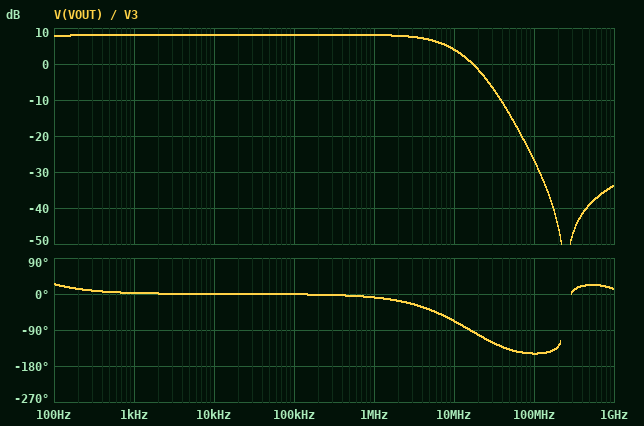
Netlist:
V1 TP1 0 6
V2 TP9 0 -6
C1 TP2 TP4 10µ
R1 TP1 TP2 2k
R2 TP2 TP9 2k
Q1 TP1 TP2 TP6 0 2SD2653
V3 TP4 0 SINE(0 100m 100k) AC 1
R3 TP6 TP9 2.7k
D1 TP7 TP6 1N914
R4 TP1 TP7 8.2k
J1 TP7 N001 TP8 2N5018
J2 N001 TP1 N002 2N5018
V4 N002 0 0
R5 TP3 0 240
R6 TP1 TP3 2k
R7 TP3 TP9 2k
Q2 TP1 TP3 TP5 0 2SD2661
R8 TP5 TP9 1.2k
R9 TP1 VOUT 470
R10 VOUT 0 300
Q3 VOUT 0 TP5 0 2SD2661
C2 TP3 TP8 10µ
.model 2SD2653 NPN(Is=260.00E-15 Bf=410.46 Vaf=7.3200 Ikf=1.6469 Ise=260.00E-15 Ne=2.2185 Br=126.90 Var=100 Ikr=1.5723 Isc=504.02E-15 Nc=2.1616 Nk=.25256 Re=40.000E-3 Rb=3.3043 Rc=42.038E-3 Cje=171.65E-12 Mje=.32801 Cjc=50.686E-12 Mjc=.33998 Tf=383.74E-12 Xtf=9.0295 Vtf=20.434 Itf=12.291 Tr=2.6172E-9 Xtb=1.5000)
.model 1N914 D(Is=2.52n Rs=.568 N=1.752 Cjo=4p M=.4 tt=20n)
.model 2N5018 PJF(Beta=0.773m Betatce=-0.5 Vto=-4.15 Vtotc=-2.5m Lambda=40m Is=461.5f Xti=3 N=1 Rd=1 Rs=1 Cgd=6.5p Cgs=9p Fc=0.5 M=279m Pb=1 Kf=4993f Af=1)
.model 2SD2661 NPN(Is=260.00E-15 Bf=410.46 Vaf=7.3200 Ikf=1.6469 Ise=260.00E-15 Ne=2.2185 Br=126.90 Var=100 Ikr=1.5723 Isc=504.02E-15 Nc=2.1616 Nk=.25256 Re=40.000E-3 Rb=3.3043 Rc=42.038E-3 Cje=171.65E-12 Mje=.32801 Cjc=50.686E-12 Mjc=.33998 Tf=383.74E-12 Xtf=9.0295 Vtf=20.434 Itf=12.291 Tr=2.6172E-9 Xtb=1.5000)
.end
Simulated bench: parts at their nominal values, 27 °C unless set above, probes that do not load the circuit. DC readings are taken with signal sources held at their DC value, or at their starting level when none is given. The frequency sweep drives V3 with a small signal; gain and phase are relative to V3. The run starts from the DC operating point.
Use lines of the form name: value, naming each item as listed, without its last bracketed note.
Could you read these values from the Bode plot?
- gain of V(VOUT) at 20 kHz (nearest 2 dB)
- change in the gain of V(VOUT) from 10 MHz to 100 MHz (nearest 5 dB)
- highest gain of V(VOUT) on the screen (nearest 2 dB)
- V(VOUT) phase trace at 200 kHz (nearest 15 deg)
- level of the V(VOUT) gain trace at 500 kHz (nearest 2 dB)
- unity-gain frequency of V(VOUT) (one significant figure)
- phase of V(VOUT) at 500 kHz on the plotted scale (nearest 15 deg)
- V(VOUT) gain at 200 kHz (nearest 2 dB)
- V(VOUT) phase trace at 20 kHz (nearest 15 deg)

gain of V(VOUT) at 20 kHz: 8 dB
change in the gain of V(VOUT) from 10 MHz to 100 MHz: -30 dB
highest gain of V(VOUT) on the screen: 8 dB
V(VOUT) phase trace at 200 kHz: 0 deg
level of the V(VOUT) gain trace at 500 kHz: 8 dB
unity-gain frequency of V(VOUT): 20 MHz
phase of V(VOUT) at 500 kHz on the plotted scale: 0 deg
V(VOUT) gain at 200 kHz: 8 dB
V(VOUT) phase trace at 20 kHz: 0 deg
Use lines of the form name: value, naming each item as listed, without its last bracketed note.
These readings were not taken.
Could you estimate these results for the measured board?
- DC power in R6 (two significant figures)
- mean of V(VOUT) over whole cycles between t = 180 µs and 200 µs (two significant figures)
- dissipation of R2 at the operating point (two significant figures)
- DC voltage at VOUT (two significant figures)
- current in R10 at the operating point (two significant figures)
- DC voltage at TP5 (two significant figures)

DC power in R6: 18 mW
mean of V(VOUT) over whole cycles between t = 180 µs and 200 µs: 2.0 V
dissipation of R2 at the operating point: 18 mW
DC voltage at VOUT: 2.0 V
current in R10 at the operating point: 6.6 mA
DC voltage at TP5: -580 mV
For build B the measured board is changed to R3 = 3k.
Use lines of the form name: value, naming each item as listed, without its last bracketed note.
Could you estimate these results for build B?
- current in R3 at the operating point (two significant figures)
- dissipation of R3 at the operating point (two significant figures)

current in R3 at the operating point: 1.8 mA
dissipation of R3 at the operating point: 9.9 mW
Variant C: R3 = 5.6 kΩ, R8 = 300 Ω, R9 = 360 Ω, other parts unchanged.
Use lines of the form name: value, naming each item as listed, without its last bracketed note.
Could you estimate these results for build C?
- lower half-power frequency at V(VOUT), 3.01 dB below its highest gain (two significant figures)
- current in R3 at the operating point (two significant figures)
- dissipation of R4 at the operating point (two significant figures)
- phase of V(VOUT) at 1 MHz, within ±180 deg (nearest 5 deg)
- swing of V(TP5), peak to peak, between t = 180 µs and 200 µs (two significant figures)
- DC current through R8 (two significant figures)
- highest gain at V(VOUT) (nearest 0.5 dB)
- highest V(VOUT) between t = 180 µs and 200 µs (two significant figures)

lower half-power frequency at V(VOUT), 3.01 dB below its highest gain: 33 Hz
current in R3 at the operating point: 980 µA
dissipation of R4 at the operating point: 4.3 mW
phase of V(VOUT) at 1 MHz, within ±180 deg: -10 deg
swing of V(TP5), peak to peak, between t = 180 µs and 200 µs: 34 mV
DC current through R8: 18 mA
highest gain at V(VOUT): 17.0 dB
highest V(VOUT) between t = 180 µs and 200 µs: 2.1 V
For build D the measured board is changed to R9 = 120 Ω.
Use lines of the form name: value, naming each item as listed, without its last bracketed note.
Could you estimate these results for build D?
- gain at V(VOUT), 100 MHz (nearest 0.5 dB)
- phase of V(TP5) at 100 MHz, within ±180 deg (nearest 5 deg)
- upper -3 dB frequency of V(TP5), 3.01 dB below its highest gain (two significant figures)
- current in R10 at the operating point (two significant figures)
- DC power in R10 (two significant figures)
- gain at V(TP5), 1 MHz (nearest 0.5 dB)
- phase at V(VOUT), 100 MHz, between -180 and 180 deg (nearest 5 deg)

gain at V(VOUT), 100 MHz: -25.5 dB
phase of V(TP5) at 100 MHz, within ±180 deg: -45 deg
upper -3 dB frequency of V(TP5), 3.01 dB below its highest gain: 8.5 MHz
current in R10 at the operating point: 14 mA
DC power in R10: 56 mW
gain at V(TP5), 1 MHz: -15.0 dB
phase at V(VOUT), 100 MHz, between -180 and 180 deg: -130 deg
